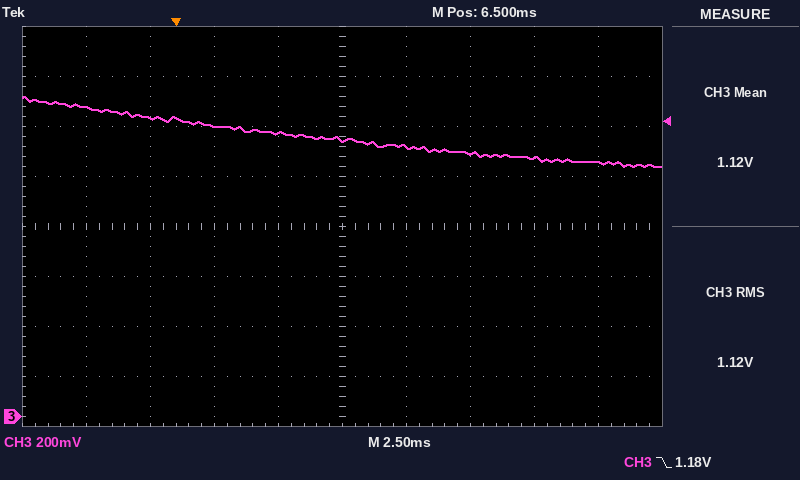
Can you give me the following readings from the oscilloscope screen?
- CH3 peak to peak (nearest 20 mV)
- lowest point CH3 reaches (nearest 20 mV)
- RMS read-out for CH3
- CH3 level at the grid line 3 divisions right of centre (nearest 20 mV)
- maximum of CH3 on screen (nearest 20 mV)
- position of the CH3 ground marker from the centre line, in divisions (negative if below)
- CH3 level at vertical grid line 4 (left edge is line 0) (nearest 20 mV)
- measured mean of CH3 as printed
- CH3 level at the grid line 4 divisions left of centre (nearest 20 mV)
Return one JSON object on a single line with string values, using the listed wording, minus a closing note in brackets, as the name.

{"CH3 peak to peak": "280 mV", "lowest point CH3 reaches": "1.00 V", "RMS read-out for CH3": "1.12 V", "CH3 level at the grid line 3 divisions right of centre": "1.04 V", "maximum of CH3 on screen": "1.28 V", "position of the CH3 ground marker from the centre line, in divisions": "-3.8 div", "CH3 level at vertical grid line 4 (left edge is line 0)": "1.14 V", "measured mean of CH3 as printed": "1.12 V", "CH3 level at the grid line 4 divisions left of centre": "1.24 V"}
